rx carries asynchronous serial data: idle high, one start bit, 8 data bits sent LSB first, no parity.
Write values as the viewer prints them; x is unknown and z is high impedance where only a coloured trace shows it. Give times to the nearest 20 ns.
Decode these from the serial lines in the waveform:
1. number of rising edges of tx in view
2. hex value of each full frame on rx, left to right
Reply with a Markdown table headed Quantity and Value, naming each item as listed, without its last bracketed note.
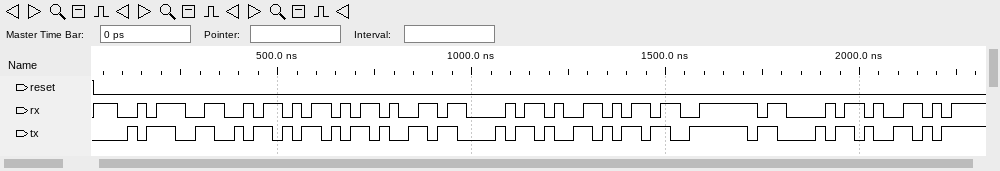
| Quantity | Value |
|---|---|
| number of rising edges of tx in view | 27 |
| hex value of each full frame on rx, left to right | 3A, 5A, 2D, 43, 59, F3, 43, 59 |
